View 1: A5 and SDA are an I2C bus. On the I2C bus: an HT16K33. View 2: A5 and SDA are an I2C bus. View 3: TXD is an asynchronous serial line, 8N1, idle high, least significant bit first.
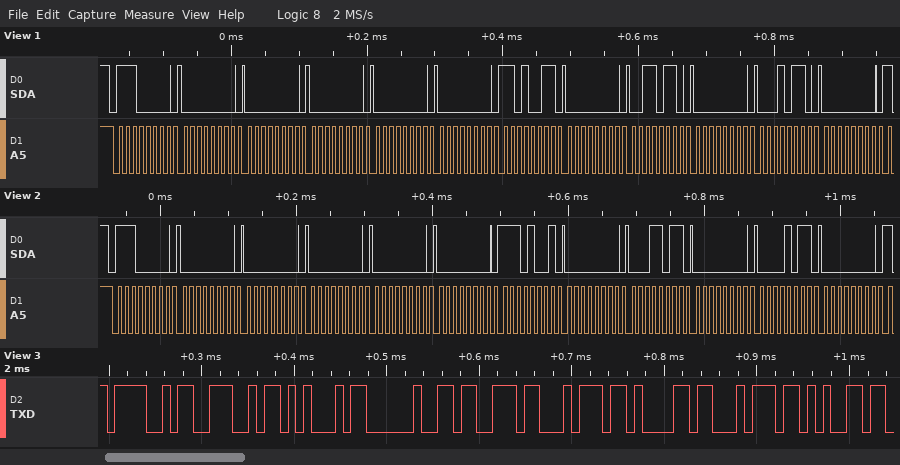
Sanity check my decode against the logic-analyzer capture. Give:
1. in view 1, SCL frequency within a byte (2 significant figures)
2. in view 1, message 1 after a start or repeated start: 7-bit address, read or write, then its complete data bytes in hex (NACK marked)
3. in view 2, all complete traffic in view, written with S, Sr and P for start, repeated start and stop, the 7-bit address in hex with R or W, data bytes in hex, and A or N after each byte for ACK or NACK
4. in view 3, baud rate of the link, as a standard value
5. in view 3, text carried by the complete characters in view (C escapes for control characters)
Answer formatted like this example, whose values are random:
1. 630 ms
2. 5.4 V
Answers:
1. 100 kHz
2. 0x70 write: 00 00 00 00 00 D3 00 36 00 16 00
3. S 70W A 00 A 00 A 00 A 00 A 00 A E9 A 00 A 1B A 00 A 0B A 00 A
4. 115200 baud
5. "ONE state"
